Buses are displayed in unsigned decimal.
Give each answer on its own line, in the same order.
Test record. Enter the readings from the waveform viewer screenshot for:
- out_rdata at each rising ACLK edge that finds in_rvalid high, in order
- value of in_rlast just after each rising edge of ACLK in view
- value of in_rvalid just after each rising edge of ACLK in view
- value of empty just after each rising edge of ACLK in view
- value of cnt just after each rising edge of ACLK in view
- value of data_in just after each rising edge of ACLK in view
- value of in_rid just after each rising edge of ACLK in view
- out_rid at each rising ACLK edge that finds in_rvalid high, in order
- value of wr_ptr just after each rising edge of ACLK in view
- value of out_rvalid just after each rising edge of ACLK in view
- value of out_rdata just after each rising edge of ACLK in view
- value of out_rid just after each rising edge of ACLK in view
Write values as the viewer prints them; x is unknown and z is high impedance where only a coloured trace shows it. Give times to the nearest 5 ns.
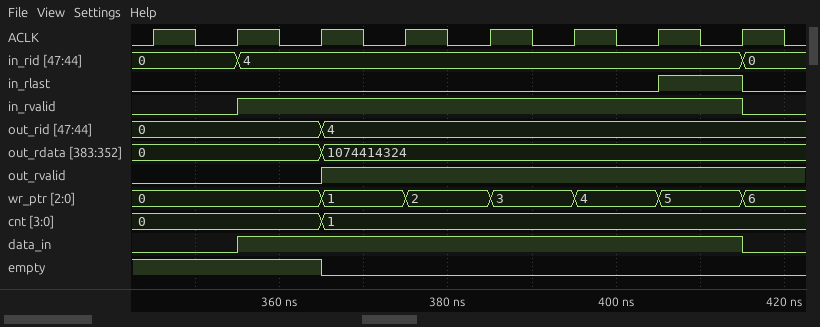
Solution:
0, 1074414324, 1074414324, 1074414324, 1074414324, 1074414324
0 0 0 0 0 0 1 0
0 1 1 1 1 1 1 0
1 1 0 0 0 0 0 0
0, 0, 1, 1, 1, 1, 1, 1
0 1 1 1 1 1 1 0
0, 4, 4, 4, 4, 4, 4, 0
0, 4, 4, 4, 4, 4
0, 0, 1, 2, 3, 4, 5, 6
0 0 1 1 1 1 1 1
0, 0, 1074414324, 1074414324, 1074414324, 1074414324, 1074414324, 1074414324
0, 0, 4, 4, 4, 4, 4, 4
